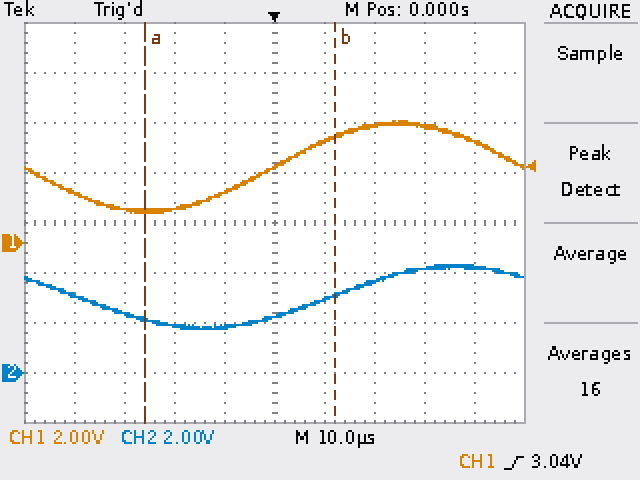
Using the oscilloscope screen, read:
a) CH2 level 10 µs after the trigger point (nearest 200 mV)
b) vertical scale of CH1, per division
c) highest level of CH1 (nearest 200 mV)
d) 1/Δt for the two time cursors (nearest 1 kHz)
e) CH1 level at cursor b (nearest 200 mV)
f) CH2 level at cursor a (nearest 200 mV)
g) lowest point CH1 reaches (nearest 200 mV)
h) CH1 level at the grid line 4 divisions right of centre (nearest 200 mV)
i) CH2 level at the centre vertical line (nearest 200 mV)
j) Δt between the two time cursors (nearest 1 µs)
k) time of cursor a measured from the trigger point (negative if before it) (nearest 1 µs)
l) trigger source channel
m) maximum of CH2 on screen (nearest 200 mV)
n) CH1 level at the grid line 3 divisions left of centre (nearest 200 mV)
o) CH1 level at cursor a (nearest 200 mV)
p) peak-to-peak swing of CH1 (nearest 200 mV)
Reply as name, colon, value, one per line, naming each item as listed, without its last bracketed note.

CH2 level 10 µs after the trigger point: 3.0 V
vertical scale of CH1, per division: 2 V
highest level of CH1: 4.8 V
1/Δt for the two time cursors: 26 kHz
CH1 level at cursor b: 4.2 V
CH2 level at cursor a: 2.2 V
lowest point CH1 reaches: 1.2 V
CH1 level at the grid line 4 divisions right of centre: 4.0 V
CH2 level at the centre vertical line: 2.2 V
Δt between the two time cursors: 38 µs
time of cursor a measured from the trigger point (negative if before it): -26 µs
trigger source channel: CH1
maximum of CH2 on screen: 4.4 V
CH1 level at the grid line 3 divisions left of centre: 1.4 V
CH1 level at cursor a: 1.2 V
peak-to-peak swing of CH1: 3.6 V
